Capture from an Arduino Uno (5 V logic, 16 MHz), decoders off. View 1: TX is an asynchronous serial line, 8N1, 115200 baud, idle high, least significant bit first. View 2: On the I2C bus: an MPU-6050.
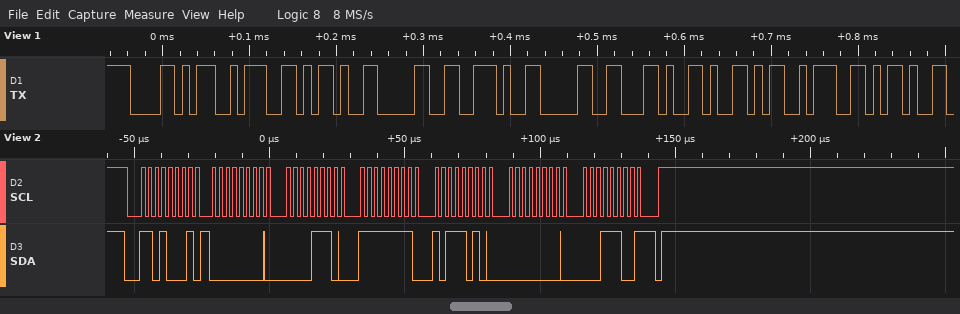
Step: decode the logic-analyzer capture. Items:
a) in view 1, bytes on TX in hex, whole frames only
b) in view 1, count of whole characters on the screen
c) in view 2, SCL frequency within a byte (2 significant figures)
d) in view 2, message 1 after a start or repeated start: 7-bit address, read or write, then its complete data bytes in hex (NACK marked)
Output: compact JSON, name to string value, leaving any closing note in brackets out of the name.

{"in view 1, bytes on TX in hex, whole frames only": "0x58 0x3A 0x2D 0x30 0x2E 0x30 0x2C 0x59 0x3A 0x2D", "in view 1, count of whole characters on the screen": "10", "in view 2, SCL frequency within a byte": "400 kHz", "in view 2, message 1 after a start or repeated start: 7-bit address, read or write, then its complete data bytes in hex": "0x68 read: 00 0E FF BA 00 1C NACK"}
